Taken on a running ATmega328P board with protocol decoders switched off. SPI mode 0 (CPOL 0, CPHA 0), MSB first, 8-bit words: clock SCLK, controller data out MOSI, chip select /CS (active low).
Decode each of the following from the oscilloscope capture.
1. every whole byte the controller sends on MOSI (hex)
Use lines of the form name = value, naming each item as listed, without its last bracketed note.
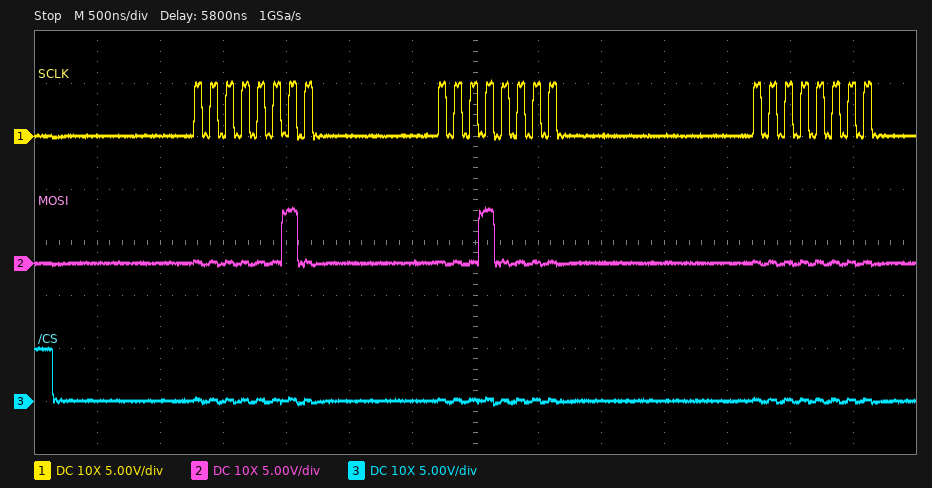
every whole byte the controller sends on MOSI = 02 10 00
